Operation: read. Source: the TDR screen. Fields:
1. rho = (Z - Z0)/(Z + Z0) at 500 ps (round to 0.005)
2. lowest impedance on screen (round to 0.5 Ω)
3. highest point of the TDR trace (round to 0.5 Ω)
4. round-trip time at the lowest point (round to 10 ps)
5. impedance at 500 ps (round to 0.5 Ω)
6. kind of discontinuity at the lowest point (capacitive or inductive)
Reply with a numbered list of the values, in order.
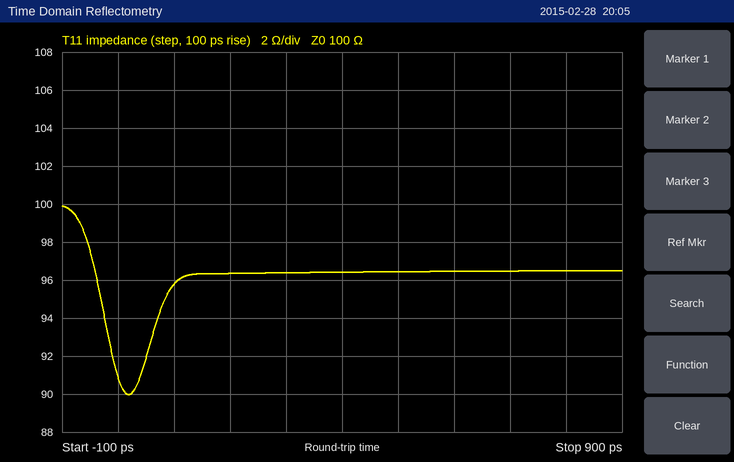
1. -0.020
2. 90.0 Ω
3. 100.0 Ω
4. 20 ps
5. 96.5 Ω
6. capacitive
